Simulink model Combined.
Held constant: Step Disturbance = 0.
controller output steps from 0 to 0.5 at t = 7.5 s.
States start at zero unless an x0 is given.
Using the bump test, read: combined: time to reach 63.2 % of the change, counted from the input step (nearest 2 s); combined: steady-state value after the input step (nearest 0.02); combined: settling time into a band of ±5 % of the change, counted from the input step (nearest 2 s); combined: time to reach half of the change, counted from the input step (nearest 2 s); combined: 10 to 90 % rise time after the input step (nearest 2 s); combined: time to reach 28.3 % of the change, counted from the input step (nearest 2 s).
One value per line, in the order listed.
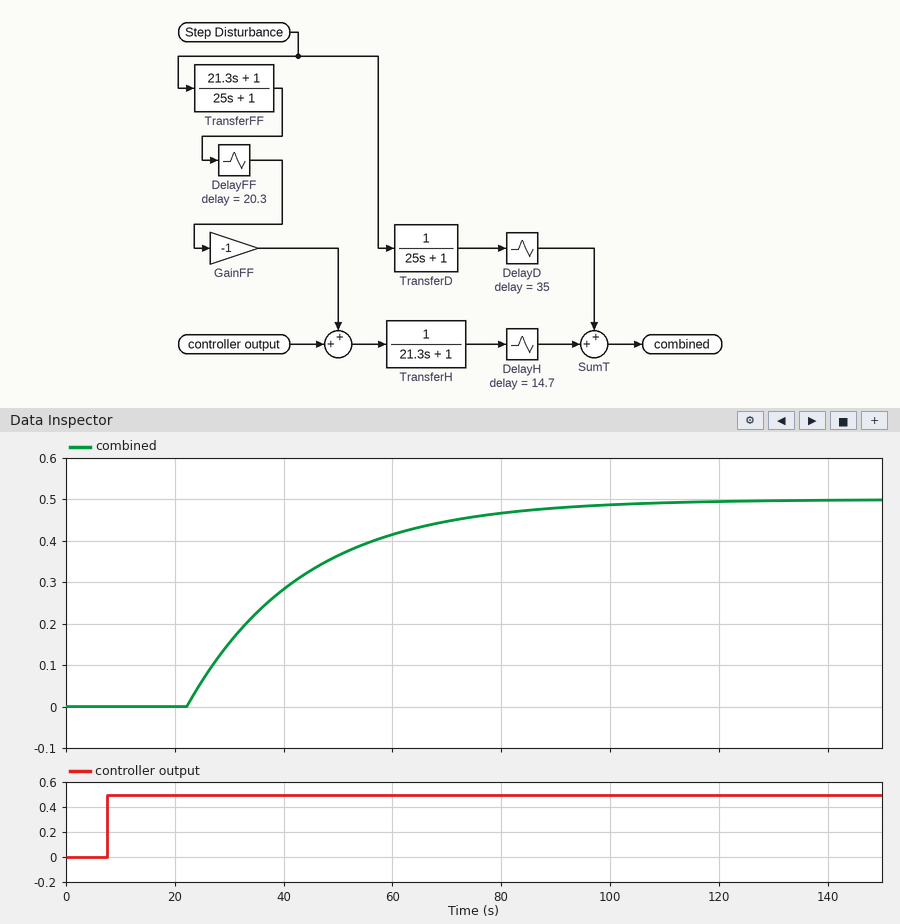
36 s
0.50
78 s
30 s
46 s
22 s
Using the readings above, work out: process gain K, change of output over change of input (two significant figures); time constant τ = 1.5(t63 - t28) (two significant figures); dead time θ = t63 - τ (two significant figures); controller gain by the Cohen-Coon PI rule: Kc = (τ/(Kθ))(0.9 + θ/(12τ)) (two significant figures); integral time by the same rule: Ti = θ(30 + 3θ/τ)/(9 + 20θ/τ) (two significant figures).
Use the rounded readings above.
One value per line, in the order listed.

1.0
21 s
15 s
1.3
21 s
